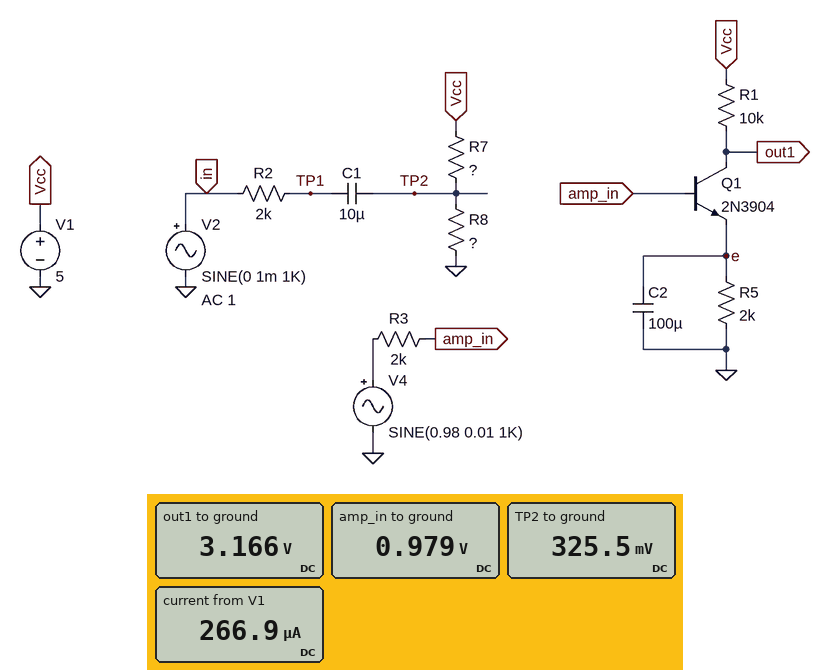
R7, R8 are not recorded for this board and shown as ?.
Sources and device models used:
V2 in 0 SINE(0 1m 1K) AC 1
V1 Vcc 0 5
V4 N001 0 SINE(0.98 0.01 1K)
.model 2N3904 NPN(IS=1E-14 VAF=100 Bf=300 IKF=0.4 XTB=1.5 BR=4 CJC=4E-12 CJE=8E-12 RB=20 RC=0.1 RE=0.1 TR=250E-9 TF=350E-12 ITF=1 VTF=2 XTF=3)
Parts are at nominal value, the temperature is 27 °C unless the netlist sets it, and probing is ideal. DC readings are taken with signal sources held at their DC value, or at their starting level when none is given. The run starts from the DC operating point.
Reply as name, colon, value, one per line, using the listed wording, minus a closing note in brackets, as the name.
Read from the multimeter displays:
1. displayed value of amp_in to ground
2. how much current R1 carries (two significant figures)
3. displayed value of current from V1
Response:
displayed value of amp_in to ground: 0.979 V
how much current R1 carries: 180 µA
displayed value of current from V1: 266.9 µA
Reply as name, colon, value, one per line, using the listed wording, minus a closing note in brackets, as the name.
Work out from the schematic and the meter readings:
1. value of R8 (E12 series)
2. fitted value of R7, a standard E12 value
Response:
value of R8: 3.9 kΩ
fitted value of R7, a standard E12 value: 56 kΩ
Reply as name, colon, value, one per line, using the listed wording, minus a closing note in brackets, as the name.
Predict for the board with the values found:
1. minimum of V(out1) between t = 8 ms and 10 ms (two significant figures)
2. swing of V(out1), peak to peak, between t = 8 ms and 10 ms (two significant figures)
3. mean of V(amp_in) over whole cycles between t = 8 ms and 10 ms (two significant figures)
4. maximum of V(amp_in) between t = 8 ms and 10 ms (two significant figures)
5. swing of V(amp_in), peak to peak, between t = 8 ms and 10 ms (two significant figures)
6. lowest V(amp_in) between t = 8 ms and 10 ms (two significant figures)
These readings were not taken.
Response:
minimum of V(out1) between t = 8 ms and 10 ms: 2.4 V
swing of V(out1), peak to peak, between t = 8 ms and 10 ms: 1.3 V
mean of V(amp_in) over whole cycles between t = 8 ms and 10 ms: 980 mV
maximum of V(amp_in) between t = 8 ms and 10 ms: 990 mV
swing of V(amp_in), peak to peak, between t = 8 ms and 10 ms: 19 mV
lowest V(amp_in) between t = 8 ms and 10 ms: 970 mV
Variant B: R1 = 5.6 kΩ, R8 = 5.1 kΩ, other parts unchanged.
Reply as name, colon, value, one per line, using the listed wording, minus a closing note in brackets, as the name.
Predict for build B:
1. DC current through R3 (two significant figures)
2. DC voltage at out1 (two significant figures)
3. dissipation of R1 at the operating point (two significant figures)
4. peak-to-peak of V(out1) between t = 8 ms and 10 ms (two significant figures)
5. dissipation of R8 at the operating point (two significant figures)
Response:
DC current through R3: 590 nA
DC voltage at out1: 4.0 V
dissipation of R1 at the operating point: 190 µW
peak-to-peak of V(out1) between t = 8 ms and 10 ms: 750 mV
dissipation of R8 at the operating point: 34 µW
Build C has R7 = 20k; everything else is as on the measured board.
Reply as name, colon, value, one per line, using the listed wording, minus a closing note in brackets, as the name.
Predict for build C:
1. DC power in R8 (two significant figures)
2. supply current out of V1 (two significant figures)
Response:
DC power in R8: 170 µW
supply current out of V1: 390 µA
